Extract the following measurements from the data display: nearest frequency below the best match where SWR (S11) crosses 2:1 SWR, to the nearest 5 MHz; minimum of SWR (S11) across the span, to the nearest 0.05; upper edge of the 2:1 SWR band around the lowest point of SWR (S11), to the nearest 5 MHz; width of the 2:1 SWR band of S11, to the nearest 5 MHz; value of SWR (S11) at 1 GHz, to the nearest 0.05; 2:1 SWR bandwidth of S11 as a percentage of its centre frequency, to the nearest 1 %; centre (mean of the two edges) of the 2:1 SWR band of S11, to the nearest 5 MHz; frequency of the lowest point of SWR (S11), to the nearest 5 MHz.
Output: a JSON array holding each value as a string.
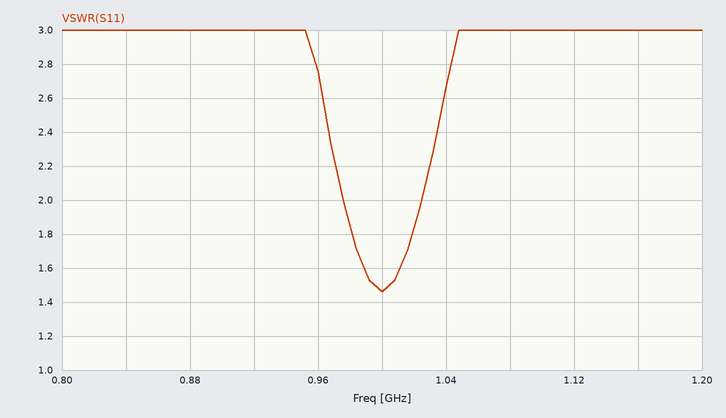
["975 MHz", "1.45", "1.025 GHz", "50 MHz", "1.45", "5 %", "1.000 GHz", "1.000 GHz"]
